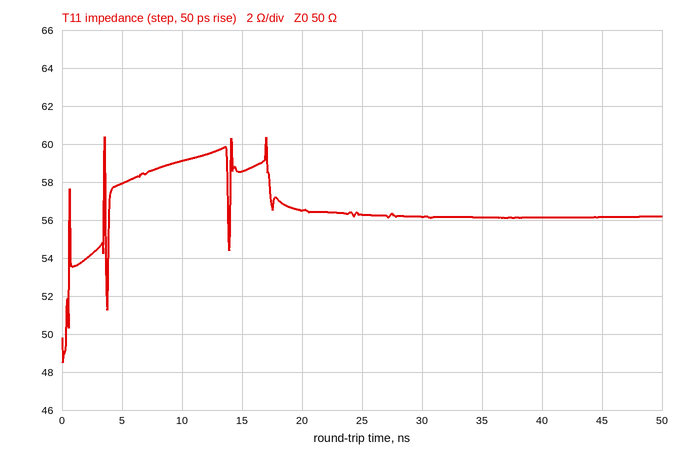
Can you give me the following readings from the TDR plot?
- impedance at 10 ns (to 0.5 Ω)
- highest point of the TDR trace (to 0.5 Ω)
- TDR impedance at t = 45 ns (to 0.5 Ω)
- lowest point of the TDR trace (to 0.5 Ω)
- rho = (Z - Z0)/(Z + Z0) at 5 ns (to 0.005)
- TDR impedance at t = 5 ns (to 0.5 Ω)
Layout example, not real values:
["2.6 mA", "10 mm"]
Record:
["59.0 Ω", "60.5 Ω", "56.0 Ω", "48.5 Ω", "+0.075", "58.0 Ω"]
